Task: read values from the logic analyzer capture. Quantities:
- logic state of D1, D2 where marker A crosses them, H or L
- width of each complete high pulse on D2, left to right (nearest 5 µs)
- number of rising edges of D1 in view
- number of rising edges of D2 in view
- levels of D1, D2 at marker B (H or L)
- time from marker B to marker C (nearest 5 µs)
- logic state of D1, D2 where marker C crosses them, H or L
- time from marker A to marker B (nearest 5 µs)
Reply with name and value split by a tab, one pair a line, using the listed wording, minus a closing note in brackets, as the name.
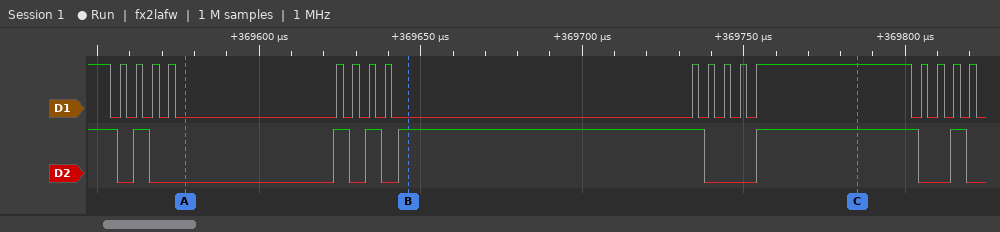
logic state of D1, D2 where marker A crosses them, H or L	D1=L, D2=L
width of each complete high pulse on D2, left to right	5 µs, 5 µs, 5 µs, 95 µs, 50 µs, 5 µs
number of rising edges of D1 in view	17
number of rising edges of D2 in view	6
levels of D1, D2 at marker B	D1=L, D2=H
time from marker B to marker C	140 µs
logic state of D1, D2 where marker C crosses them, H or L	D1=H, D2=H
time from marker A to marker B	70 µs
